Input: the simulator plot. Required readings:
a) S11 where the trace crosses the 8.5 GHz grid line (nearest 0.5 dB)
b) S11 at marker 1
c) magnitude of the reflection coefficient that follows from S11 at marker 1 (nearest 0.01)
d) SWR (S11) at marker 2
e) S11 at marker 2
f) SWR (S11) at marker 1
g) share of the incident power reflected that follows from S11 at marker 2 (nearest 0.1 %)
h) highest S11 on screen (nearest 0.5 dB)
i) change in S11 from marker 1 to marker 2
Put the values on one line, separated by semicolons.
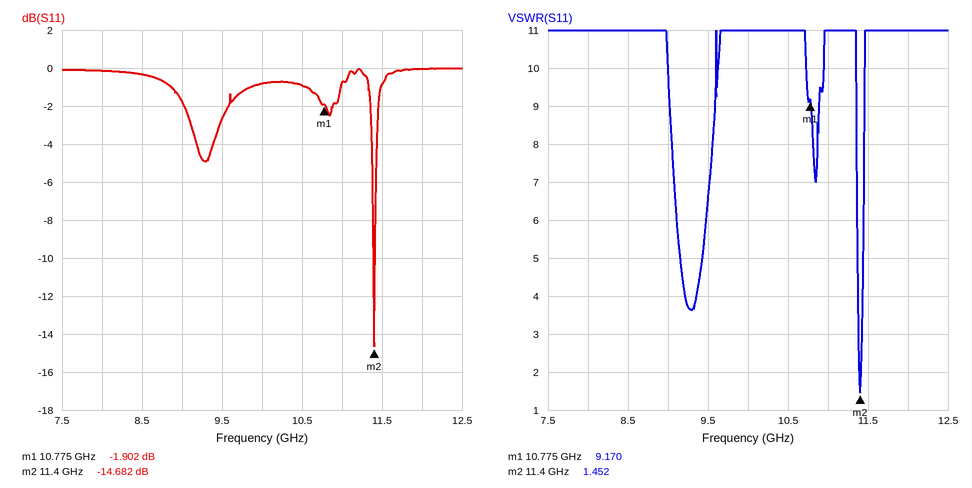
-0.5 dB; -1.902 dB; 0.80; 1.452; -14.682 dB; 9.170; 3.4 %; 0.0 dB; -12.780 dB
